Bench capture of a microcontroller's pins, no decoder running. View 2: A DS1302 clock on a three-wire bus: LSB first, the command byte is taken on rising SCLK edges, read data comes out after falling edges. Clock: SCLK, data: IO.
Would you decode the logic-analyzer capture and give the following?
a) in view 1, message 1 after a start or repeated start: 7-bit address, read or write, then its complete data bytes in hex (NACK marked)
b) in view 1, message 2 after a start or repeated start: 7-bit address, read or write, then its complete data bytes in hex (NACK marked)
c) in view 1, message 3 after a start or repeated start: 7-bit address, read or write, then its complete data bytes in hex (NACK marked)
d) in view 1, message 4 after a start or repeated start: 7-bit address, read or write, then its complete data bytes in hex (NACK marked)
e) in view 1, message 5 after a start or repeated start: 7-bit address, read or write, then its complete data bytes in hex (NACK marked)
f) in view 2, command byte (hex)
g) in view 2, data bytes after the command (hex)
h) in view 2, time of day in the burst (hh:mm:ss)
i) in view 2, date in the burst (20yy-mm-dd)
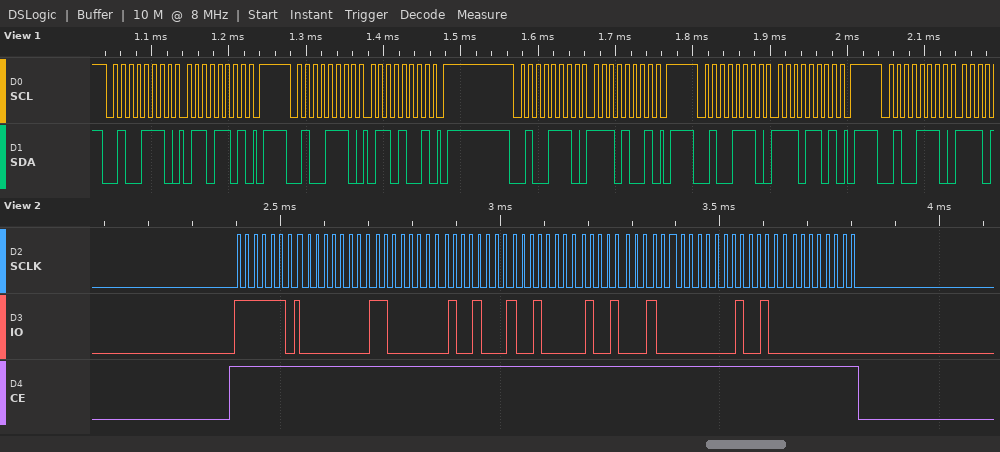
0x27 write: 6D
0x27 write: 69
0x27 write: E9
0x27 write: ED
0x27 write
0xBF
00 03 12 09 12 01 24 00
12:03:00
2024-12-09
